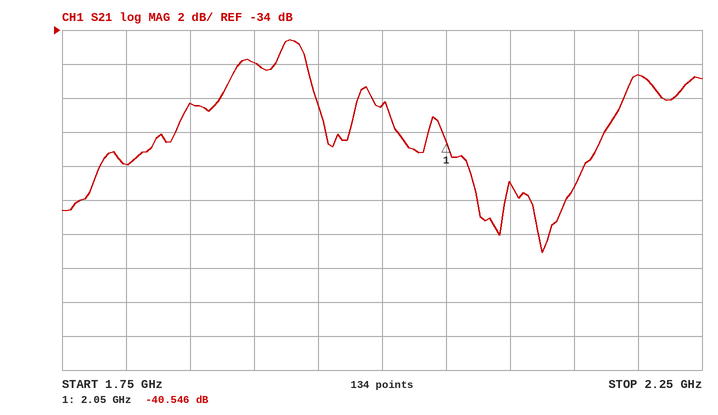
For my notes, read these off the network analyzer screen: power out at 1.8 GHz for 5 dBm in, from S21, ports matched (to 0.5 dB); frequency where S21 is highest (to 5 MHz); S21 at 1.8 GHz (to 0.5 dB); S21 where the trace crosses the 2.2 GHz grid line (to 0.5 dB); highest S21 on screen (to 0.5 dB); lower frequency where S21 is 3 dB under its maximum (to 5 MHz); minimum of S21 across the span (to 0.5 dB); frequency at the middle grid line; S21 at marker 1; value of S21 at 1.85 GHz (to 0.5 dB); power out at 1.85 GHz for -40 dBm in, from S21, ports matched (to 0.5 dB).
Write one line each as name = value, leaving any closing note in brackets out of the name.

power out at 1.8 GHz for 5 dBm in, from S21, ports matched = -37.0 dBm
frequency where S21 is highest = 1.930 GHz
S21 at 1.8 GHz = -42.0 dB
S21 where the trace crosses the 2.2 GHz grid line = -36.5 dB
highest S21 on screen = -34.5 dB
lower frequency where S21 is 3 dB under its maximum = 1.875 GHz
minimum of S21 across the span = -47.0 dB
frequency at the middle grid line = 2 GHz
S21 at marker 1 = -40.546 dB
value of S21 at 1.85 GHz = -38.5 dB
power out at 1.85 GHz for -40 dBm in, from S21, ports matched = -78.5 dBm
